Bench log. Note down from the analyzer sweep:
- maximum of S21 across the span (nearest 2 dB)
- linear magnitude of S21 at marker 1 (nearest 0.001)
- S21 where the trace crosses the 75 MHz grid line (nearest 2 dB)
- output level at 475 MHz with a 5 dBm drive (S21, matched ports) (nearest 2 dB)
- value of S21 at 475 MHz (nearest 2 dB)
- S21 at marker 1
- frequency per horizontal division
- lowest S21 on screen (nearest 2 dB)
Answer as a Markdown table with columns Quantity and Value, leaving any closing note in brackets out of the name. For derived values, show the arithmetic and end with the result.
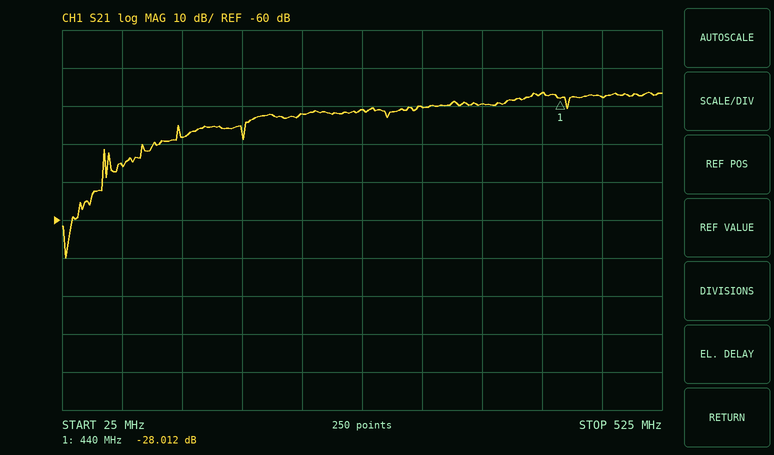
| Quantity | Value |
|---|---|
| maximum of S21 across the span | -26 dB |
| linear magnitude of S21 at marker 1 | 10^(-28.012/20) ≈ 0.040 |
| S21 where the trace crosses the 75 MHz grid line | -46 dB |
| output level at 475 MHz with a 5 dBm drive (S21, matched ports) | 5 dBm + (-28 dB) = -22 dBm |
| value of S21 at 475 MHz | -28 dB |
| S21 at marker 1 | -28.012 dB |
| frequency per horizontal division | 50 MHz |
| lowest S21 on screen | -70 dB |
